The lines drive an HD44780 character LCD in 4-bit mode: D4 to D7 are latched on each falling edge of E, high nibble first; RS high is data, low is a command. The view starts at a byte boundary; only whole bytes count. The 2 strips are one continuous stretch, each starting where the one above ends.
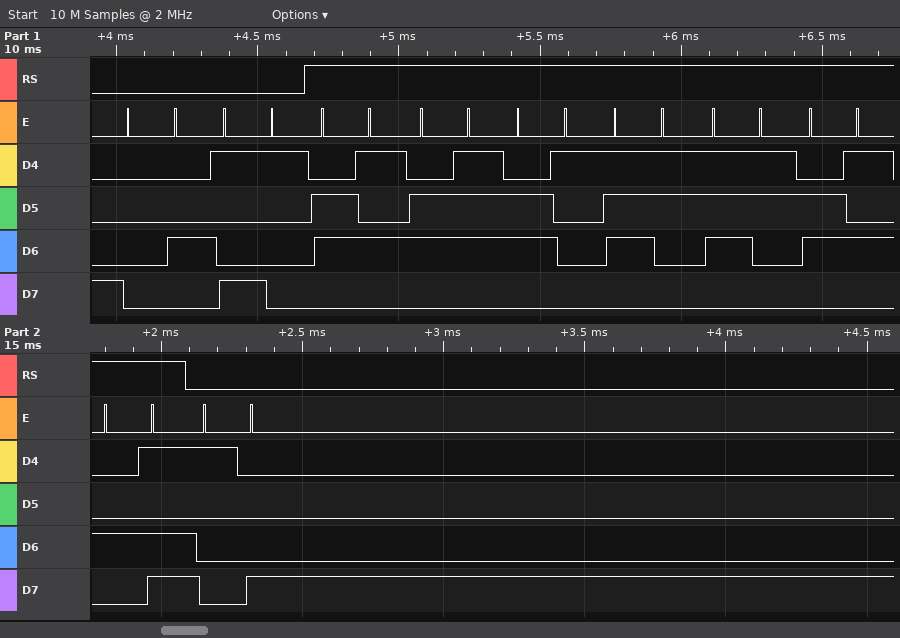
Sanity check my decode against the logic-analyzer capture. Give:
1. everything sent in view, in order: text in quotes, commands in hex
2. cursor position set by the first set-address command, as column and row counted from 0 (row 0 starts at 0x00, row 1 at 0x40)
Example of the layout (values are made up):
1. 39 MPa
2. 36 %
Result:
1. 0x04 0x91 "egasseM" 0x18
2. column 17, row 0
